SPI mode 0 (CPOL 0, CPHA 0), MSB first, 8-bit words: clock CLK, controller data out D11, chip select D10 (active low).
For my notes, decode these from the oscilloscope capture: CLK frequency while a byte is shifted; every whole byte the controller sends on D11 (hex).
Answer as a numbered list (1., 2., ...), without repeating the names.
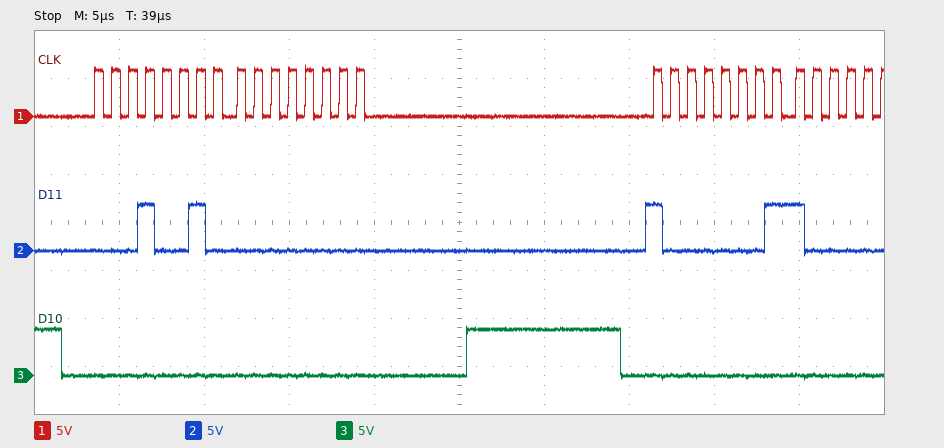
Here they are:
1. 1 MHz
2. 0x12 0x00 0x81
